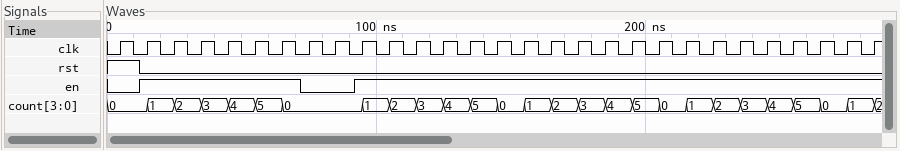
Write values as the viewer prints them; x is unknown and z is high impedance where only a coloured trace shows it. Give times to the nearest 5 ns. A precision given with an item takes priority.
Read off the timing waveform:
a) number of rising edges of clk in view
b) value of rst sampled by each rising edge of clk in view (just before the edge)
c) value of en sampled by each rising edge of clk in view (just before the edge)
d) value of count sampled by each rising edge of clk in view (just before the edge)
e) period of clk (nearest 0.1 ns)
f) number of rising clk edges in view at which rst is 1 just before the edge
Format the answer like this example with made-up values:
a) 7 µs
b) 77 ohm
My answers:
a) 29
b) 1 0 0 0 0 0 0 0 0 0 0 0 0 0 0 0 0 0 0 0 0 0 0 0 0 0 0 0 0
c) 0 1 1 1 1 1 1 0 0 1 1 1 1 1 1 1 1 1 1 1 1 1 1 1 1 1 1 1 1
d) 0, 0, 1, 2, 3, 4, 5, 0, 0, 0, 1, 2, 3, 4, 5, 0, 1, 2, 3, 4, 5, 0, 1, 2, 3, 4, 5, 0, 1
e) 10 ns
f) 1
